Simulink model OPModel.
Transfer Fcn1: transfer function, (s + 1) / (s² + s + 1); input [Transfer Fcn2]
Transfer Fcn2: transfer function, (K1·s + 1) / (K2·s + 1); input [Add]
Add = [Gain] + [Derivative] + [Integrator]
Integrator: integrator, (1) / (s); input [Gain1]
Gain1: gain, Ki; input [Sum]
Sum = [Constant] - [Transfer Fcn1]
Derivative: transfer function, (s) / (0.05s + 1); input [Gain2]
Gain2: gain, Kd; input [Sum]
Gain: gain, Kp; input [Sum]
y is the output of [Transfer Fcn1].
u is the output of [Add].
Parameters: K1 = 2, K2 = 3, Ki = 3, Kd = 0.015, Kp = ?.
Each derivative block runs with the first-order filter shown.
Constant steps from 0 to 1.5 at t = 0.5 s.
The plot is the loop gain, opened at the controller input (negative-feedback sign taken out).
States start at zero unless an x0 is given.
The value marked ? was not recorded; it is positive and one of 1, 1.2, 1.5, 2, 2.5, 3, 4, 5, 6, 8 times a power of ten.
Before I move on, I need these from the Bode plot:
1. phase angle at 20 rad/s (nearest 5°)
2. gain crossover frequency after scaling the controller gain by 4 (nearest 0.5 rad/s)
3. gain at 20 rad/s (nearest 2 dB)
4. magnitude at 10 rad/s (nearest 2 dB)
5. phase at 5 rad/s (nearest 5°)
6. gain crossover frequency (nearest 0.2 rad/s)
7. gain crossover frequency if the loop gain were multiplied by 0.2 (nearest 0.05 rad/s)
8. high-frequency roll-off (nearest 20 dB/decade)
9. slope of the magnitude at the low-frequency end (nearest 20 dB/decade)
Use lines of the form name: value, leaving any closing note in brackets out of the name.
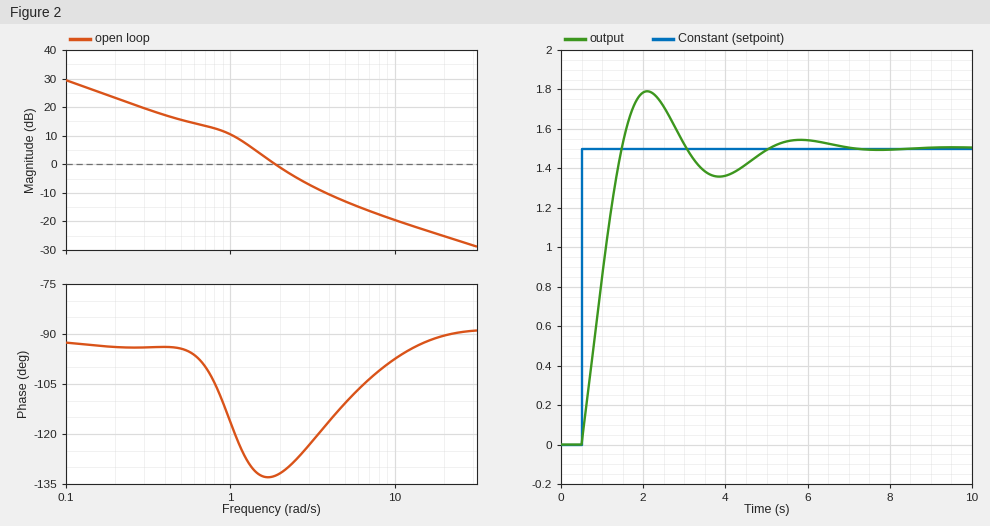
phase angle at 20 rad/s: -90°
gain crossover frequency after scaling the controller gain by 4: 4.5 rad/s
gain at 20 rad/s: -26 dB
magnitude at 10 rad/s: -20 dB
phase at 5 rad/s: -110°
gain crossover frequency: 1.8 rad/s
gain crossover frequency if the loop gain were multiplied by 0.2: 0.65 rad/s
high-frequency roll-off: -20 dB/decade
slope of the magnitude at the low-frequency end: -20 dB/decade
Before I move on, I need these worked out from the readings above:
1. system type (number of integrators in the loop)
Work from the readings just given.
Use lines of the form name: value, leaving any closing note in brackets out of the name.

system type: 1
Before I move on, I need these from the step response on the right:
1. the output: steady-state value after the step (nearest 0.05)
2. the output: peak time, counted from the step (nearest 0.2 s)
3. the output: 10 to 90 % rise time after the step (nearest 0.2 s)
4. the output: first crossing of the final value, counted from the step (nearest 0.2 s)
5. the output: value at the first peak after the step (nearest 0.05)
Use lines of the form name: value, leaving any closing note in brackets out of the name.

the output: steady-state value after the step: 1.50
the output: peak time, counted from the step: 1.6 s
the output: 10 to 90 % rise time after the step: 0.8 s
the output: first crossing of the final value, counted from the step: 1.0 s
the output: value at the first peak after the step: 1.80
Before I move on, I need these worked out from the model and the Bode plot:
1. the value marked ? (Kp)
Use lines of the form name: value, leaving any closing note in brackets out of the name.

the value marked ?: 1.5
